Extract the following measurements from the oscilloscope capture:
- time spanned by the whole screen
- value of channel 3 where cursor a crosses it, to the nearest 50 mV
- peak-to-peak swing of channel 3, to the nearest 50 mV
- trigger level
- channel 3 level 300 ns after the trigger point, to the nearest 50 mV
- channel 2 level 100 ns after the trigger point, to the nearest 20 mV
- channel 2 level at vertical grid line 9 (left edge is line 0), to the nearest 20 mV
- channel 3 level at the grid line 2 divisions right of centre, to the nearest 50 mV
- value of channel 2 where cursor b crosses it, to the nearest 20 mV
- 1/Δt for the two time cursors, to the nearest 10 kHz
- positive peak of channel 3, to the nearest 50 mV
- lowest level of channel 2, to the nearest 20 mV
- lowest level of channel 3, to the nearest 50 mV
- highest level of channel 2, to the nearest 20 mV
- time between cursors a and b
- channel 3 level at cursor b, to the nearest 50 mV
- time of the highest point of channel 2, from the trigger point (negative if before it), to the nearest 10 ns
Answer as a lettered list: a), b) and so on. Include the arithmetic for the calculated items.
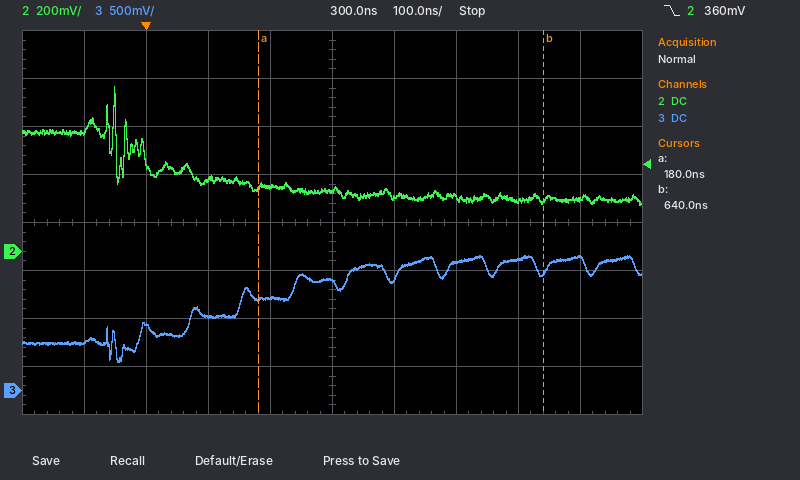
a) 1 µs
b) 950 mV
c) 1.40 V − (300 mV) = 1.10 V
d) 360 mV
e) 1.15 V
f) 300 mV
g) 220 mV
h) 1.35 V
i) 220 mV
j) 1 / 460 ns ≈ 2.17 MHz
k) 1.40 V
l) 200 mV
m) 300 mV
n) 680 mV
o) 640 ns − (180 ns) = 460 ns
p) 1.25 V
q) -50 ns
